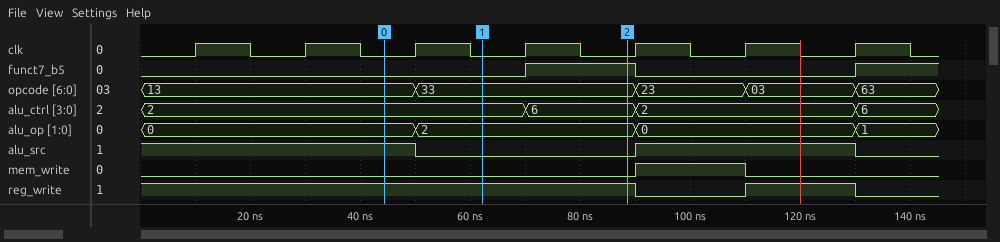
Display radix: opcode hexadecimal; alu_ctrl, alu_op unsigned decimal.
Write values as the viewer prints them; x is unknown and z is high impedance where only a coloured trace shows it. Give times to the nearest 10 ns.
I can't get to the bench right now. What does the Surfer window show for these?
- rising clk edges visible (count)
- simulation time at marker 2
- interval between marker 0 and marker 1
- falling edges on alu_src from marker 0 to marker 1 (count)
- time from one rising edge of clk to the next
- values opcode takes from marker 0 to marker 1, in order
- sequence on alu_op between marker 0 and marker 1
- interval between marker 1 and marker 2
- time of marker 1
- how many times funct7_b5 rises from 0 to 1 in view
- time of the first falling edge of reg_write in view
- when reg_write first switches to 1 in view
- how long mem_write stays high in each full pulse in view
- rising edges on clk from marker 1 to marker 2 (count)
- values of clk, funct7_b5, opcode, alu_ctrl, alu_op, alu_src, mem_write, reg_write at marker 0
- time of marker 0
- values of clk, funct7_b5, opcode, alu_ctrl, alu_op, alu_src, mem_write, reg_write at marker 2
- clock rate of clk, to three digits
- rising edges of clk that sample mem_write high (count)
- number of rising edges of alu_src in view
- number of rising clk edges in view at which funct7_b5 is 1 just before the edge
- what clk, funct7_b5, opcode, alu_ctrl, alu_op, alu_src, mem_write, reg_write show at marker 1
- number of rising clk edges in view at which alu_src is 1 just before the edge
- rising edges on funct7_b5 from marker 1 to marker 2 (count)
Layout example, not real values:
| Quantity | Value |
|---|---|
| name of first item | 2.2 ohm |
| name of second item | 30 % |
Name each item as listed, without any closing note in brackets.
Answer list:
| Quantity | Value |
|---|---|
| rising clk edges visible | 7 |
| simulation time at marker 2 | 90 ns |
| interval between marker 0 and marker 1 | 20 ns |
| falling edges on alu_src from marker 0 to marker 1 | 1 |
| time from one rising edge of clk to the next | 20 ns |
| values opcode takes from marker 0 to marker 1, in order | 13, 33 |
| sequence on alu_op between marker 0 and marker 1 | 0, 2 |
| interval between marker 1 and marker 2 | 30 ns |
| time of marker 1 | 60 ns |
| how many times funct7_b5 rises from 0 to 1 in view | 2 |
| time of the first falling edge of reg_write in view | 90 ns |
| when reg_write first switches to 1 in view | 110 ns |
| how long mem_write stays high in each full pulse in view | 20 ns |
| rising edges on clk from marker 1 to marker 2 | 1 |
| values of clk, funct7_b5, opcode, alu_ctrl, alu_op, alu_src, mem_write, reg_write at marker 0 | clk=0, funct7_b5=0, opcode=13, alu_ctrl=2, alu_op=0, alu_src=1, mem_write=0, reg_write=1 |
| time of marker 0 | 40 ns |
| values of clk, funct7_b5, opcode, alu_ctrl, alu_op, alu_src, mem_write, reg_write at marker 2 | clk=0, funct7_b5=1, opcode=33, alu_ctrl=6, alu_op=2, alu_src=0, mem_write=0, reg_write=1 |
| clock rate of clk, to three digits | 50.0 MHz |
| rising edges of clk that sample mem_write high | 1 |
| number of rising edges of alu_src in view | 1 |
| number of rising clk edges in view at which funct7_b5 is 1 just before the edge | 1 |
| what clk, funct7_b5, opcode, alu_ctrl, alu_op, alu_src, mem_write, reg_write show at marker 1 | clk=0, funct7_b5=0, opcode=33, alu_ctrl=2, alu_op=2, alu_src=0, mem_write=0, reg_write=1 |
| number of rising clk edges in view at which alu_src is 1 just before the edge | 5 |
| rising edges on funct7_b5 from marker 1 to marker 2 | 1 |
